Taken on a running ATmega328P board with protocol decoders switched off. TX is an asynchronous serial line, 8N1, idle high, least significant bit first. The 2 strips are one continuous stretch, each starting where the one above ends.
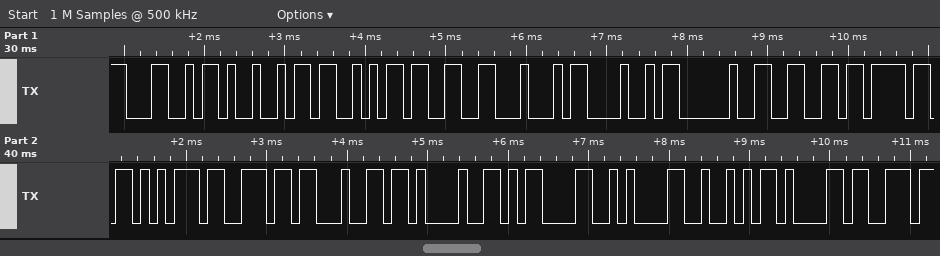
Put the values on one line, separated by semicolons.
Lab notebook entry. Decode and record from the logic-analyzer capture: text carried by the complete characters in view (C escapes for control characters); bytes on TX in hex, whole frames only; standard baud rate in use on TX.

"LIS3DH found!\r\nRa"; 4C 49 53 33 44 48 20 66 6F 75 6E 64 21 0D 0A 52 61; 9600 baud
